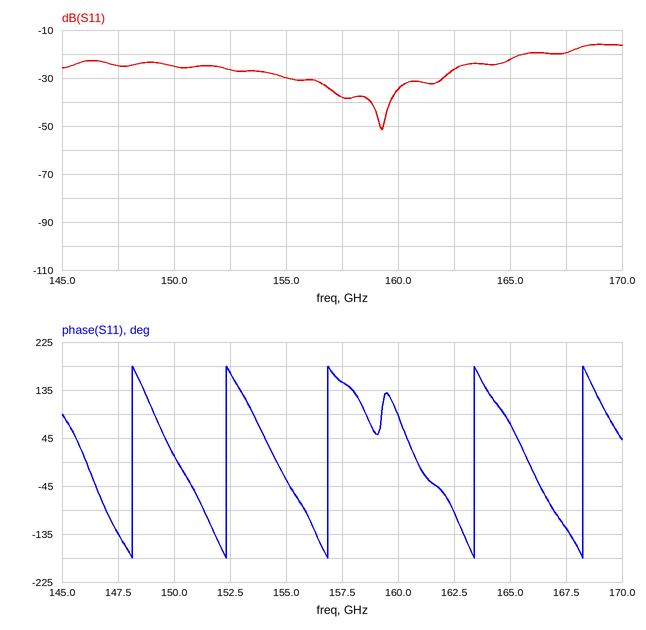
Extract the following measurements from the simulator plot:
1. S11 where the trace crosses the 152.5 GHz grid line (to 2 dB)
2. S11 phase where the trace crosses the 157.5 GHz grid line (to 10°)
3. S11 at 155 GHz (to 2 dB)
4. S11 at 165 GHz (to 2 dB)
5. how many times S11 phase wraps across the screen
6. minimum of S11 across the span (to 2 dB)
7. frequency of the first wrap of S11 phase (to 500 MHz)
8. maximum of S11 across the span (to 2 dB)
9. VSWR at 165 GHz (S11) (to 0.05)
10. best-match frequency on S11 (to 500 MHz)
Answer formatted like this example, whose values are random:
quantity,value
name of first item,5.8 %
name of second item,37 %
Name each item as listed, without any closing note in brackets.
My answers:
quantity,value
S11 where the trace crosses the 152.5 GHz grid line,-26 dB
S11 phase where the trace crosses the 157.5 GHz grid line,150°
S11 at 155 GHz,-30 dB
S11 at 165 GHz,-22 dB
how many times S11 phase wraps across the screen,5
minimum of S11 across the span,-52 dB
frequency of the first wrap of S11 phase,148.0 GHz
maximum of S11 across the span,-16 dB
VSWR at 165 GHz (S11),1.15
best-match frequency on S11,159.5 GHz
